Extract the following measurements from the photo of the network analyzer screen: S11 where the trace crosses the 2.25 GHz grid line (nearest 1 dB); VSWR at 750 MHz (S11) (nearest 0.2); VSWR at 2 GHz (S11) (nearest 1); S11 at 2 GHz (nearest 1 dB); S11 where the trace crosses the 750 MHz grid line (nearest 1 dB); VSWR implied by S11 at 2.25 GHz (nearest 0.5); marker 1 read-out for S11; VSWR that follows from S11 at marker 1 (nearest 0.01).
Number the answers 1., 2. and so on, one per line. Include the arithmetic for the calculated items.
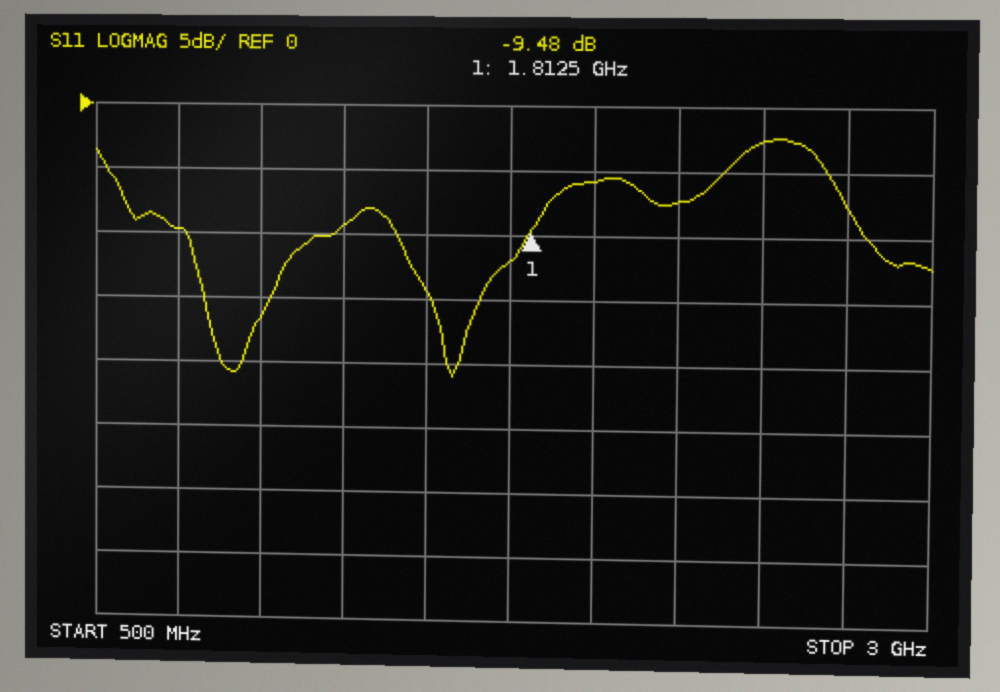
1. -7 dB
2. |Γ| = 10^(-10/20) = 0.3162; VSWR = (1 + 0.3162)/(1 − 0.3162) ≈ 1.92, so 2.0 to the nearest 0.2
3. |Γ| = 10^(-6/20) = 0.5012; VSWR = (1 + 0.5012)/(1 − 0.5012) ≈ 3
4. -6 dB
5. -10 dB
6. |Γ| = 10^(-7/20) = 0.4467; VSWR = (1 + 0.4467)/(1 − 0.4467) ≈ 2.61, so 2.5 to the nearest 0.5
7. -9.48 dB
8. (1 + 0.3357)/(1 − 0.3357) ≈ 2.01
